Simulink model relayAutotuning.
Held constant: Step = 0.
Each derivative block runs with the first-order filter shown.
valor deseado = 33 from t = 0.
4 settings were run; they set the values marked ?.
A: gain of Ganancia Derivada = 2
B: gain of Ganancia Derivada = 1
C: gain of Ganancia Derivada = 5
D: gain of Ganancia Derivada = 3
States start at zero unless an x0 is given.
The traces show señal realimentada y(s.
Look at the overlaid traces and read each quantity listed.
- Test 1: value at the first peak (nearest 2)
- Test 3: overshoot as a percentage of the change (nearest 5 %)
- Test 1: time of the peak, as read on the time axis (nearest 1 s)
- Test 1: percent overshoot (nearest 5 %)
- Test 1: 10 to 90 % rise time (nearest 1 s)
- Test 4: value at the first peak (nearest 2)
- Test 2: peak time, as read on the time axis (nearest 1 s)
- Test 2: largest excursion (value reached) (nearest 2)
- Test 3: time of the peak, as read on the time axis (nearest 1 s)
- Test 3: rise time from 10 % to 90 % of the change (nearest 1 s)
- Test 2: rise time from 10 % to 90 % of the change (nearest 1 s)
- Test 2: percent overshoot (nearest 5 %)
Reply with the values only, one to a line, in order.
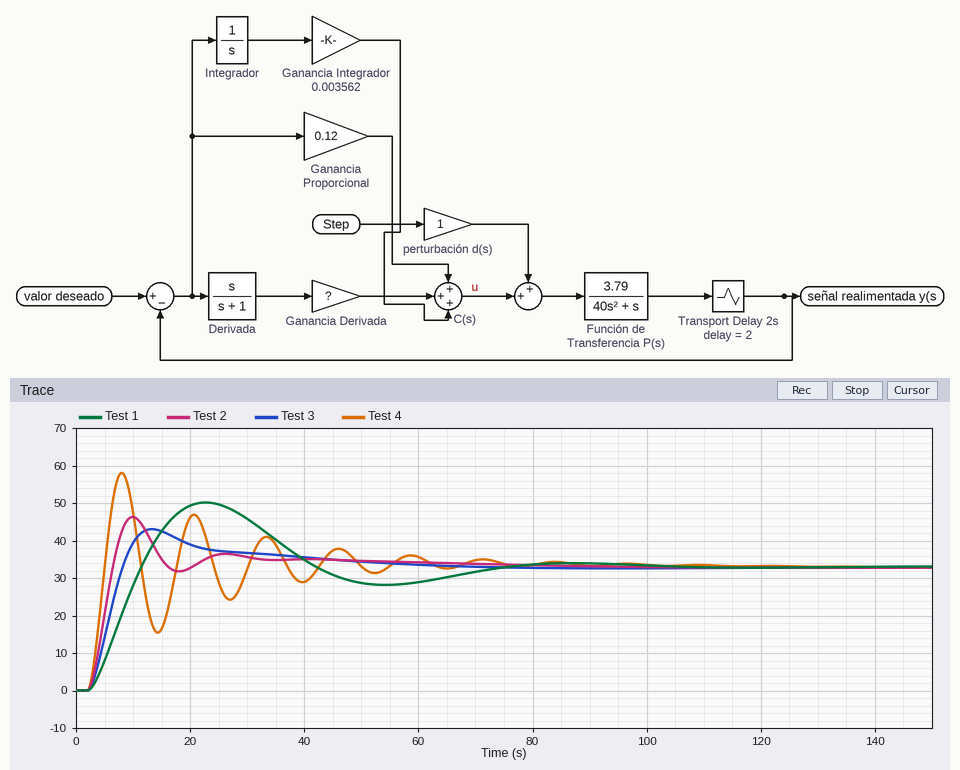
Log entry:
50
30 %
23 s
50 %
7 s
58
10 s
46
13 s
4 s
3 s
40 %
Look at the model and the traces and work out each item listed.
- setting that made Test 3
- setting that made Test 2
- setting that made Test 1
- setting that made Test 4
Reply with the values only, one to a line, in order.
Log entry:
A
D
B
C
